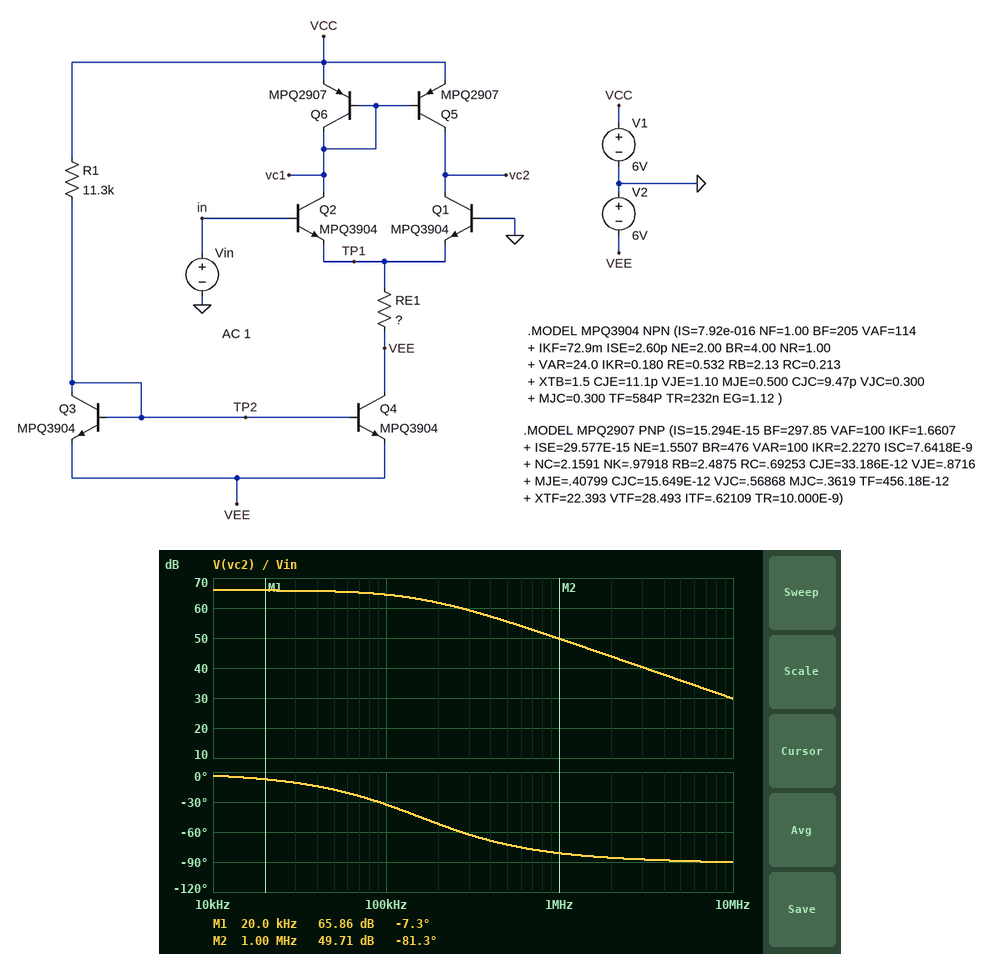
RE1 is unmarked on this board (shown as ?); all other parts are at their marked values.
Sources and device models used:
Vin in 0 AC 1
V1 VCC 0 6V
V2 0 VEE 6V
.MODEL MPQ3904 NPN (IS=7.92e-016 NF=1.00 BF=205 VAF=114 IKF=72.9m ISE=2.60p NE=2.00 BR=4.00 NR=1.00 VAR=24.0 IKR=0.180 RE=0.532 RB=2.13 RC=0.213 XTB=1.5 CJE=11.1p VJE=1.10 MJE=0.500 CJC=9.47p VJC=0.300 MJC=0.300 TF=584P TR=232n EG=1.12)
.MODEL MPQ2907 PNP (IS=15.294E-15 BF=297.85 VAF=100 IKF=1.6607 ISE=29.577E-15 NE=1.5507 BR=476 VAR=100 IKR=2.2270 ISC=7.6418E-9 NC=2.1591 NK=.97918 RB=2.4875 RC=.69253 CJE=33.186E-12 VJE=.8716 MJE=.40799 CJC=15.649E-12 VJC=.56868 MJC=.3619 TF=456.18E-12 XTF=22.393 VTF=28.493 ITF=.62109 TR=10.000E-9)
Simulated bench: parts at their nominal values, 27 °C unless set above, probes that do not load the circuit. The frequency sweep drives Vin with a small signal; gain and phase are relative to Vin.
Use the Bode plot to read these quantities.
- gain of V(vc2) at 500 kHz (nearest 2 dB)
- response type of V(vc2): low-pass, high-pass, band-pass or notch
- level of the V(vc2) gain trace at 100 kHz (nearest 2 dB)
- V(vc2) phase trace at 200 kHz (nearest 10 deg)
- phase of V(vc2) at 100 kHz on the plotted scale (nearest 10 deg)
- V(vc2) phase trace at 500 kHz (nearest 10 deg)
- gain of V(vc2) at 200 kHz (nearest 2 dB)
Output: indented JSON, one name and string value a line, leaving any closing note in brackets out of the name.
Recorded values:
{
  "gain of V(vc2) at 500 kHz": "56 dB",
  "response type of V(vc2): low-pass, high-pass, band-pass or notch": "low-pass",
  "level of the V(vc2) gain trace at 100 kHz": "64 dB",
  "V(vc2) phase trace at 200 kHz": "-50 deg",
  "phase of V(vc2) at 100 kHz on the plotted scale": "-30 deg",
  "V(vc2) phase trace at 500 kHz": "-70 deg",
  "gain of V(vc2) at 200 kHz": "62 dB"
}
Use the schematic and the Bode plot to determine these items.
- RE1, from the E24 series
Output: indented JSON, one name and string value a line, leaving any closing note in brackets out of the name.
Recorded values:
{
  "RE1, from the E24 series": "1.5 kΩ"
}
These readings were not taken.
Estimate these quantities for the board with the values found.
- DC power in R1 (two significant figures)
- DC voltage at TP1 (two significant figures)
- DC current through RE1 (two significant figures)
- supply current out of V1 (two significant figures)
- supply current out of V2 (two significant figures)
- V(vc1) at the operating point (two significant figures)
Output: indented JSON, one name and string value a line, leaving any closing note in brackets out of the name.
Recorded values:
{
  "DC power in R1": "11 mW",
  "DC voltage at TP1": "-740 mV",
  "DC current through RE1": "3.5 mA",
  "supply current out of V1": "4.5 mA",
  "supply current out of V2": "4.5 mA",
  "V(vc1) at the operating point": "5.3 V"
}
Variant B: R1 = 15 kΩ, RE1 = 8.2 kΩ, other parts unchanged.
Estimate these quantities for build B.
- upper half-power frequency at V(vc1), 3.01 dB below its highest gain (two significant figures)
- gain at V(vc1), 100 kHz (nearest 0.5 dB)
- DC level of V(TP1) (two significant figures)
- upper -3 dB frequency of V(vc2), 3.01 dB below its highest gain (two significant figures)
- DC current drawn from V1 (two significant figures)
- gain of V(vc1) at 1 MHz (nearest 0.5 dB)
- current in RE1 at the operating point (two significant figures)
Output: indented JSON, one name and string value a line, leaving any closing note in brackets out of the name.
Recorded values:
{
  "upper half-power frequency at V(vc1), 3.01 dB below its highest gain": "34 kHz",
  "gain at V(vc1), 100 kHz": "-19.5 dB",
  "DC level of V(TP1)": "-690 mV",
  "upper -3 dB frequency of V(vc2), 3.01 dB below its highest gain": "31 kHz",
  "DC current drawn from V1": "1.4 mA",
  "gain of V(vc1) at 1 MHz": "-22.5 dB",
  "current in RE1 at the operating point": "650 µA"
}
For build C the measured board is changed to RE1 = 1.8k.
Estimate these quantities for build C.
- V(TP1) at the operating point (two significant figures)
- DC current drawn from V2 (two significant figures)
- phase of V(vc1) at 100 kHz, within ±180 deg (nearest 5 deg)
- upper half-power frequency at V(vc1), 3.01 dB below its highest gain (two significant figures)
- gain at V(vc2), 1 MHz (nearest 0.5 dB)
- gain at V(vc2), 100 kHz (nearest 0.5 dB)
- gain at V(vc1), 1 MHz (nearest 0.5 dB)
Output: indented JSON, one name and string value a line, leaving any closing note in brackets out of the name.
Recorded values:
{
  "V(TP1) at the operating point": "-730 mV",
  "DC current drawn from V2": "3.9 mA",
  "phase of V(vc1) at 100 kHz, within ±180 deg": "155 deg",
  "upper half-power frequency at V(vc1), 3.01 dB below its highest gain": "150 kHz",
  "gain at V(vc2), 1 MHz": "48.5 dB",
  "gain at V(vc2), 100 kHz": "64.0 dB",
  "gain at V(vc1), 1 MHz": "-20.5 dB"
}
